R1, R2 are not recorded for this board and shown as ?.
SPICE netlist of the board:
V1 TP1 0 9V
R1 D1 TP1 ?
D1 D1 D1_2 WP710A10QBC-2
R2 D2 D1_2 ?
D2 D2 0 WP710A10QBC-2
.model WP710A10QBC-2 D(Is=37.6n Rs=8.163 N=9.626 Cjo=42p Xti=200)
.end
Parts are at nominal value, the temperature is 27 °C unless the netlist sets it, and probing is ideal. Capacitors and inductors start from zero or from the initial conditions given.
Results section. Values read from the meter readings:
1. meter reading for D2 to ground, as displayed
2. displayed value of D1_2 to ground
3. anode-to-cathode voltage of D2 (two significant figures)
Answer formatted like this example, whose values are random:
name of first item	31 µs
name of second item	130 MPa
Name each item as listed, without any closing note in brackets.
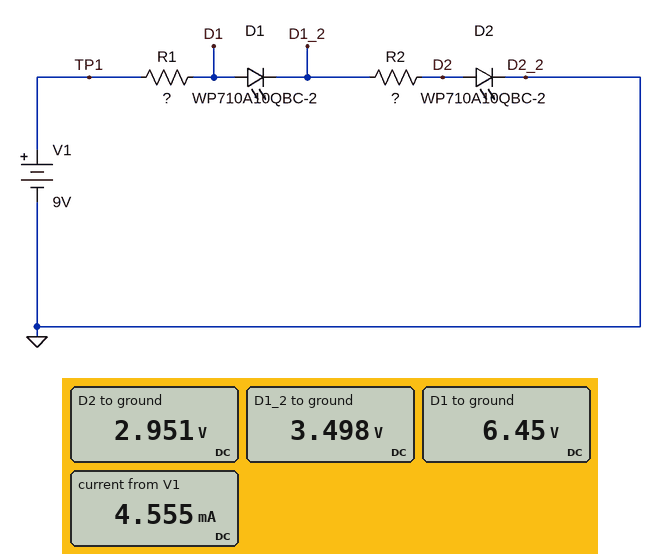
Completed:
meter reading for D2 to ground, as displayed	2.951 V
displayed value of D1_2 to ground	3.498 V
anode-to-cathode voltage of D2	3.0 V
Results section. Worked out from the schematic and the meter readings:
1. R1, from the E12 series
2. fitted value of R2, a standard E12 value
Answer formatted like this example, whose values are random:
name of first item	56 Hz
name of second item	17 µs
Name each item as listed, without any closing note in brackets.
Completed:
R1, from the E12 series	560 Ω
fitted value of R2, a standard E12 value	120 Ω
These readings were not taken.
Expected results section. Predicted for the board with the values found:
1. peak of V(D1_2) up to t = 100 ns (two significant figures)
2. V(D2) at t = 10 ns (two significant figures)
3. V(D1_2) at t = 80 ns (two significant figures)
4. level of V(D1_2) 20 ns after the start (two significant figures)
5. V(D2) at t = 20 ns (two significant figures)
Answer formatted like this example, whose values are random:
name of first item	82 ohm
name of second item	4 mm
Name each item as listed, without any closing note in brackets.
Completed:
peak of V(D1_2) up to t = 100 ns	3.5 V
V(D2) at t = 10 ns	1.5 V
V(D1_2) at t = 80 ns	3.5 V
level of V(D1_2) 20 ns after the start	2.9 V
V(D2) at t = 20 ns	2.1 V
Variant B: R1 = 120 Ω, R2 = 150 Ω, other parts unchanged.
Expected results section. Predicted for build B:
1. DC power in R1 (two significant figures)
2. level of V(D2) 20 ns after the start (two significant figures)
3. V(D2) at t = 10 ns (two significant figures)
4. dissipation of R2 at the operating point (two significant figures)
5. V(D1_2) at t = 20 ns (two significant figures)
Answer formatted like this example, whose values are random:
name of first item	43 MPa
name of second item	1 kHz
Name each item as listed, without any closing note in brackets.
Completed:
DC power in R1	11 mW
level of V(D2) 20 ns after the start	3.0 V
V(D2) at t = 10 ns	2.3 V
dissipation of R2 at the operating point	14 mW
V(D1_2) at t = 20 ns	4.7 V
